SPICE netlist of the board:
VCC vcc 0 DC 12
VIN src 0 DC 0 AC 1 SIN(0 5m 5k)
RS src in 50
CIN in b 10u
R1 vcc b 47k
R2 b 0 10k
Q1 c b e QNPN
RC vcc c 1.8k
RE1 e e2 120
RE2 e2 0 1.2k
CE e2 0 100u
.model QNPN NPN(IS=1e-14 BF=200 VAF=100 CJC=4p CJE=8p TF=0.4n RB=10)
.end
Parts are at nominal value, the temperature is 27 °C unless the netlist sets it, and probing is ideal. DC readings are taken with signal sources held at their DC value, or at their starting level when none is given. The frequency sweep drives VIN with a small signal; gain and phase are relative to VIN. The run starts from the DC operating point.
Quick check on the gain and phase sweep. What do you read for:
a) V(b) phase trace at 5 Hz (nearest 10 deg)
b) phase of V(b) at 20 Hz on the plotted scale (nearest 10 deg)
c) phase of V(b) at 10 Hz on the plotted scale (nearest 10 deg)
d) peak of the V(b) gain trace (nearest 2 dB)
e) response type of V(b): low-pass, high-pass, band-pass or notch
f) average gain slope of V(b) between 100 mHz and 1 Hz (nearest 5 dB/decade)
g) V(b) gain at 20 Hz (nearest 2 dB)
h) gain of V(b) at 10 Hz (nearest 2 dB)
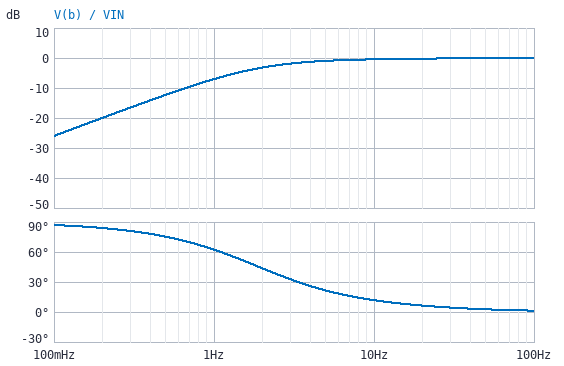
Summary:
20 deg
10 deg
10 deg
0 dB
high-pass
20 dB/decade
0 dB
0 dB
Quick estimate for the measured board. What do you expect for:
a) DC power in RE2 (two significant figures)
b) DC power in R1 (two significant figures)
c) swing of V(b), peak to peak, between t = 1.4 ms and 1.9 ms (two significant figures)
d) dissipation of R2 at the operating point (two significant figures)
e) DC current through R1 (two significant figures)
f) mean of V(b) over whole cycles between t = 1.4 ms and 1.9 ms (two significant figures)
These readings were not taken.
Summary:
1.4 mW
2.1 mW
9.9 mV
430 µW
210 µA
2.1 V
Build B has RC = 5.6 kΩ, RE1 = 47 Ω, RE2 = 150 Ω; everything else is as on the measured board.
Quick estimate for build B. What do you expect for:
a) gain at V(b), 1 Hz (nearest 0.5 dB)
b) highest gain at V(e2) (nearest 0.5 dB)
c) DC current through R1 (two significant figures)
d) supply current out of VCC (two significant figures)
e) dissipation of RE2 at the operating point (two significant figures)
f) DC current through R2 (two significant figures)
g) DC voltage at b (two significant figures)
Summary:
-37.0 dB
-21.5 dB
230 µA
2.3 mA
710 µW
110 µA
1.1 V
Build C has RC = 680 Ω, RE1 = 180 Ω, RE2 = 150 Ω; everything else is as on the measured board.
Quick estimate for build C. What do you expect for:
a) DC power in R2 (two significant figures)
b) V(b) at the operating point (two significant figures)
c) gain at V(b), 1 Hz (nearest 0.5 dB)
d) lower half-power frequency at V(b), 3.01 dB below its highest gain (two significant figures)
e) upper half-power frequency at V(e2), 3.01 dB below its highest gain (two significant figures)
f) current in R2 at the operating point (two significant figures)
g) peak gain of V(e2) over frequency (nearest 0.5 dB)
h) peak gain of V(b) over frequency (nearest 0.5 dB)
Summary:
380 µW
2.0 V
-7.5 dB
2.2 Hz
23 Hz
200 µA
-8.0 dB
0 dB
